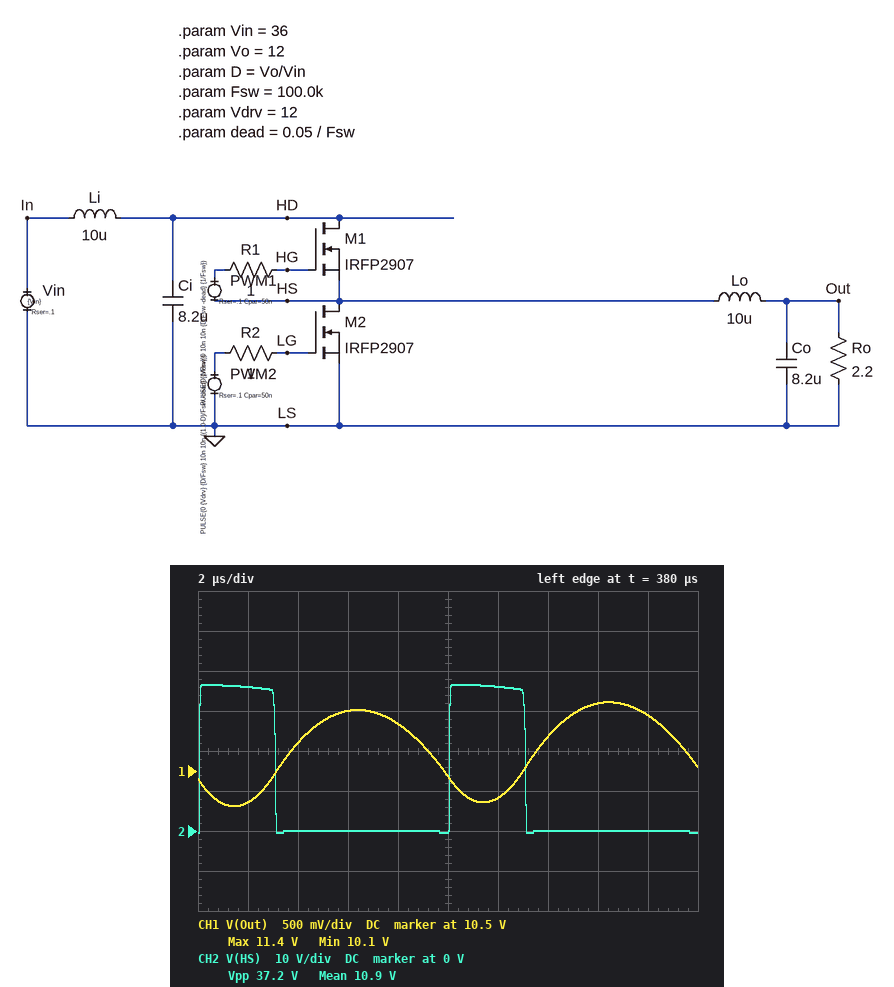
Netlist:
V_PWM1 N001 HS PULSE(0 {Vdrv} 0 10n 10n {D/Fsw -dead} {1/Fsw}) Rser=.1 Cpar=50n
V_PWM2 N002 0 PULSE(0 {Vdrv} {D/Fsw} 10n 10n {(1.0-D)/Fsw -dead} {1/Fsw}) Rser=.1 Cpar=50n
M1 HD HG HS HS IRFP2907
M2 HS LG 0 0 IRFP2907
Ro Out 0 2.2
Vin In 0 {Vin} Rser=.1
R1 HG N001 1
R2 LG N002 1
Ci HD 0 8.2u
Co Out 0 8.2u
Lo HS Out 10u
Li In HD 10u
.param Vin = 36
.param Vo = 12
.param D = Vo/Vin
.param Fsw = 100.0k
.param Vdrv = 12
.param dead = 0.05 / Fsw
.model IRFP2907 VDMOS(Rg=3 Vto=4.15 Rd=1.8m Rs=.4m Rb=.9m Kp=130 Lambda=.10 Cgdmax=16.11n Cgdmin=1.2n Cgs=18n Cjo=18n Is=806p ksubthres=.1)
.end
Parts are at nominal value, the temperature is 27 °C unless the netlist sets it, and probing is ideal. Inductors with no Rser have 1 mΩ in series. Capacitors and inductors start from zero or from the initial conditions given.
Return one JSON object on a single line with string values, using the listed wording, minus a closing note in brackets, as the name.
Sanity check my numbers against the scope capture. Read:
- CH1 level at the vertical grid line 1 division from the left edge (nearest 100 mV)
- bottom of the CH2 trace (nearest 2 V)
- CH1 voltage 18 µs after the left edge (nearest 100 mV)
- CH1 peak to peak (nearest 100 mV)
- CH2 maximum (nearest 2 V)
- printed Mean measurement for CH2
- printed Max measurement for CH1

{"CH1 level at the vertical grid line 1 division from the left edge": "10.1 V", "bottom of the CH2 trace": "0 V", "CH1 voltage 18 µs after the left edge": "11.2 V", "CH1 peak to peak": "1.3 V", "CH2 maximum": "36 V", "printed Mean measurement for CH2": "10.9 V", "printed Max measurement for CH1": "11.4 V"}
